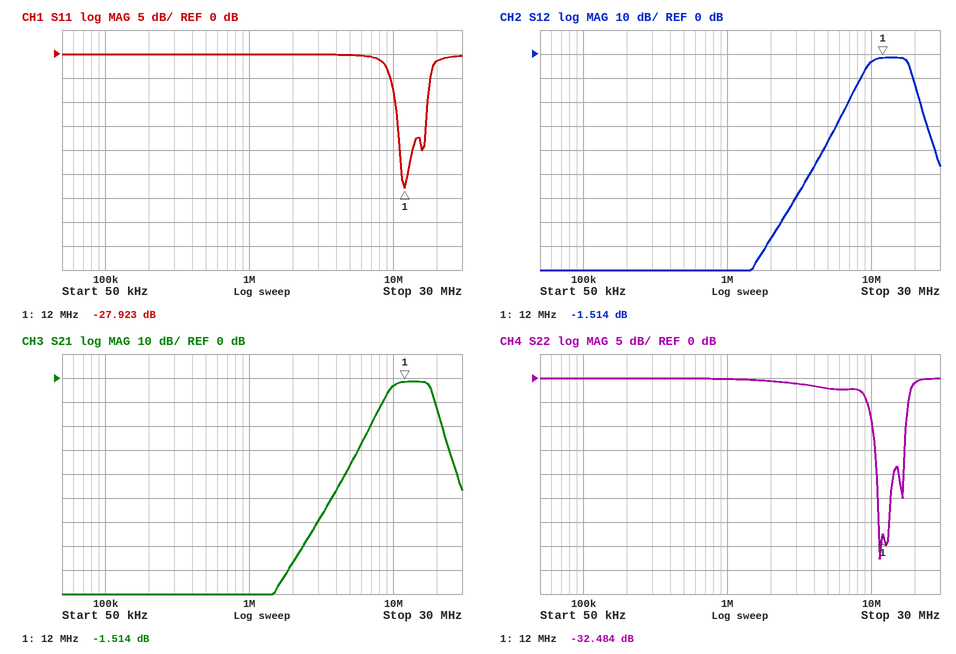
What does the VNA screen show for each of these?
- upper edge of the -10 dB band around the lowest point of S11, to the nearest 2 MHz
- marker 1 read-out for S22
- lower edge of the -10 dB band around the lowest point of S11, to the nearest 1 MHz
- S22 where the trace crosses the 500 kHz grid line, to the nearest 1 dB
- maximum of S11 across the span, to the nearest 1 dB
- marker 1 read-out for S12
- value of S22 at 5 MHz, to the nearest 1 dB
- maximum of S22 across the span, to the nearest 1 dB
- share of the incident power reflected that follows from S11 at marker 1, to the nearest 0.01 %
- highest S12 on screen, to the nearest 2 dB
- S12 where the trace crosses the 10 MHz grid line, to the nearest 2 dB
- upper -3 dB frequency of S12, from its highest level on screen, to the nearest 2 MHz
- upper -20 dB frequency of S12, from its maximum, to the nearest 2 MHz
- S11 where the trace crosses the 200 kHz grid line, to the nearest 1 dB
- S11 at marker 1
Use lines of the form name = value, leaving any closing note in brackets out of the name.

upper edge of the -10 dB band around the lowest point of S11, to the nearest 2 MHz = 18 MHz
marker 1 read-out for S22 = -32.484 dB
lower edge of the -10 dB band around the lowest point of S11, to the nearest 1 MHz = 10 MHz
S22 where the trace crosses the 500 kHz grid line, to the nearest 1 dB = 0 dB
maximum of S11 across the span, to the nearest 1 dB = 0 dB
marker 1 read-out for S12 = -1.514 dB
value of S22 at 5 MHz, to the nearest 1 dB = -2 dB
maximum of S22 across the span, to the nearest 1 dB = 0 dB
share of the incident power reflected that follows from S11 at marker 1, to the nearest 0.01 % = 0.16 %
highest S12 on screen, to the nearest 2 dB = -2 dB
S12 where the trace crosses the 10 MHz grid line, to the nearest 2 dB = -4 dB
upper -3 dB frequency of S12, from its highest level on screen, to the nearest 2 MHz = 18 MHz
upper -20 dB frequency of S12, from its maximum, to the nearest 2 MHz = 22 MHz
S11 where the trace crosses the 200 kHz grid line, to the nearest 1 dB = 0 dB
S11 at marker 1 = -27.923 dB
